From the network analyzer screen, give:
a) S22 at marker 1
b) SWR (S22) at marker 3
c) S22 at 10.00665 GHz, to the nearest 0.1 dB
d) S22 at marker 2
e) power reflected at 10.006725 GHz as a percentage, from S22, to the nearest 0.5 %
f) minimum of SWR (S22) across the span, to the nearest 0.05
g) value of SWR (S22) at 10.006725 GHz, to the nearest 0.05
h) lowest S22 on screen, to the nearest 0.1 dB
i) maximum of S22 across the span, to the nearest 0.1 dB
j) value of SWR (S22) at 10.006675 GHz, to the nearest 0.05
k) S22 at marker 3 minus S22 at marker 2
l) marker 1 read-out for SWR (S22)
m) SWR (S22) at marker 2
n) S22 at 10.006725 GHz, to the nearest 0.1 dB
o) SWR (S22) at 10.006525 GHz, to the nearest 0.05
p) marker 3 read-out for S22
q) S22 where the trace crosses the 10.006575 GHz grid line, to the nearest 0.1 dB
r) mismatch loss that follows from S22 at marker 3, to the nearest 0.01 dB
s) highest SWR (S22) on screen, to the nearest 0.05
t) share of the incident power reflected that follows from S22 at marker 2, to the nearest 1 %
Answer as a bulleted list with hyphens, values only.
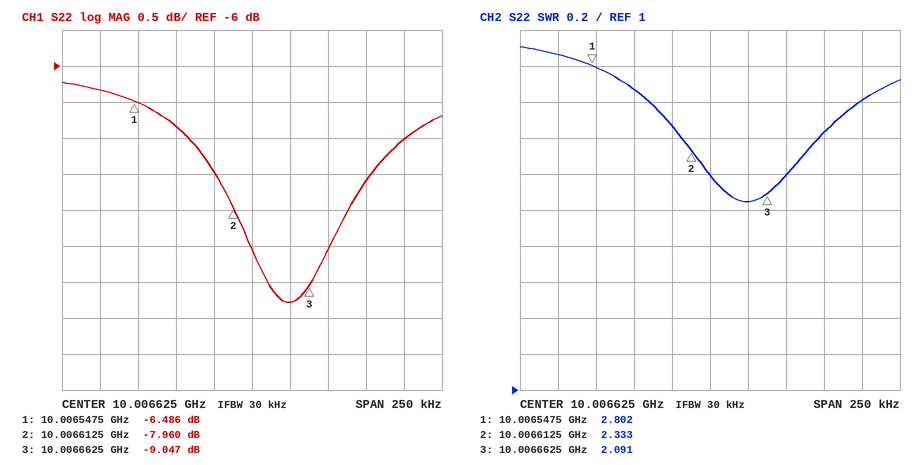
- -6.486 dB
- 2.091
- -9.3 dB
- -7.960 dB
- 20.0 %
- 2.05
- 2.60
- -9.3 dB
- -6.2 dB
- 2.20
- -1.087 dB
- 2.802
- 2.333
- -7.0 dB
- 2.85
- -9.047 dB
- -6.8 dB
- 0.58 dB
- 2.90
- 16 %
